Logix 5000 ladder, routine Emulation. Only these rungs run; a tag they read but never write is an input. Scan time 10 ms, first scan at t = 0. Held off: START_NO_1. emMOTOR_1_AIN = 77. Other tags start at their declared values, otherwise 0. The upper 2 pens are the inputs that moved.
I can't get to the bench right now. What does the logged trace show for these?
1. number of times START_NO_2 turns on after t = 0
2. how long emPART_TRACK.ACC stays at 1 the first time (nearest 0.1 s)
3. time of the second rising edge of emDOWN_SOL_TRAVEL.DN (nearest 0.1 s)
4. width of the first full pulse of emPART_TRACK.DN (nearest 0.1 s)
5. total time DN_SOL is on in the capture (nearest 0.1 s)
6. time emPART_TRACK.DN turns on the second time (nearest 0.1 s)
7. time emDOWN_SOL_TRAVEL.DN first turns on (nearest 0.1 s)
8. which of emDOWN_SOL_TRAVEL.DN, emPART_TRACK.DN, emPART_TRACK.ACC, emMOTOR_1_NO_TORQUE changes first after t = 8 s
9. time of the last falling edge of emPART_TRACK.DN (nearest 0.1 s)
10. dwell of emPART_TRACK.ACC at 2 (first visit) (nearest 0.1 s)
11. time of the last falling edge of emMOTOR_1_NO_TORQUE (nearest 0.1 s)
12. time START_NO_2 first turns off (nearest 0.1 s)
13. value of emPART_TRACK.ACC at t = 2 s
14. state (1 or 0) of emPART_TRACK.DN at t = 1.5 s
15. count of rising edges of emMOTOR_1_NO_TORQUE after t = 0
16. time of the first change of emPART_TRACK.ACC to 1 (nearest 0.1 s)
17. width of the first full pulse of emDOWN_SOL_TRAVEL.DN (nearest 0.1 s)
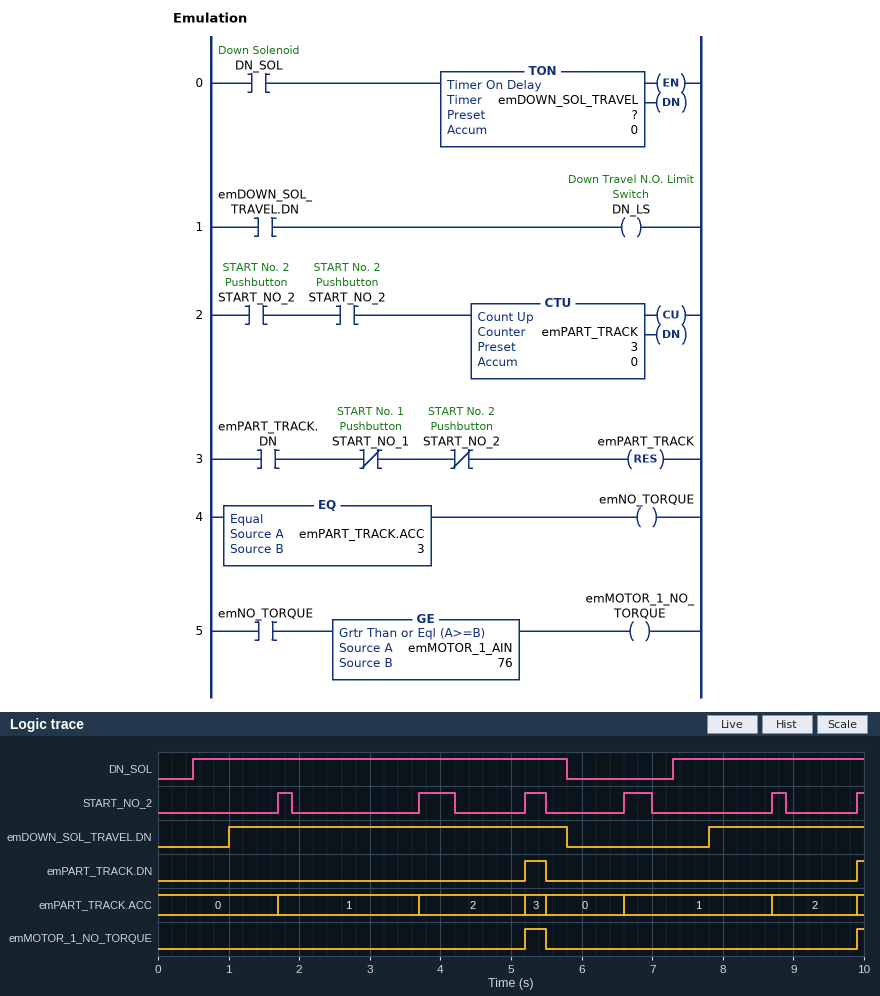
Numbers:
6
2.0 s
7.8 s
0.3 s
8.0 s
9.9 s
1.0 s
emPART_TRACK.ACC
5.5 s
1.5 s
5.5 s
1.9 s
1
0
2
1.7 s
4.8 s
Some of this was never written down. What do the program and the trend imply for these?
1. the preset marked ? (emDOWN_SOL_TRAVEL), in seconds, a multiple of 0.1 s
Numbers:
0.5 s
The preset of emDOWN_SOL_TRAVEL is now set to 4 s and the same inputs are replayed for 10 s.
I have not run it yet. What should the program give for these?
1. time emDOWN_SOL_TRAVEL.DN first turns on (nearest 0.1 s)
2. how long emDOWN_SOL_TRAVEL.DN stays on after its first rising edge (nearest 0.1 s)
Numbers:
4.5 s
1.3 s
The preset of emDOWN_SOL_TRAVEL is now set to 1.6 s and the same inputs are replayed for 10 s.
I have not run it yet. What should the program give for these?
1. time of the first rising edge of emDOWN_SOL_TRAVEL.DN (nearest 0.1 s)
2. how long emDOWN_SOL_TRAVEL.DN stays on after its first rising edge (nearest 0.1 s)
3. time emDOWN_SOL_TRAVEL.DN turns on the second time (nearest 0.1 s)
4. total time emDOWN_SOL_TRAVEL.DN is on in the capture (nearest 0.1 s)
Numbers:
2.1 s
3.7 s
8.9 s
4.8 s
